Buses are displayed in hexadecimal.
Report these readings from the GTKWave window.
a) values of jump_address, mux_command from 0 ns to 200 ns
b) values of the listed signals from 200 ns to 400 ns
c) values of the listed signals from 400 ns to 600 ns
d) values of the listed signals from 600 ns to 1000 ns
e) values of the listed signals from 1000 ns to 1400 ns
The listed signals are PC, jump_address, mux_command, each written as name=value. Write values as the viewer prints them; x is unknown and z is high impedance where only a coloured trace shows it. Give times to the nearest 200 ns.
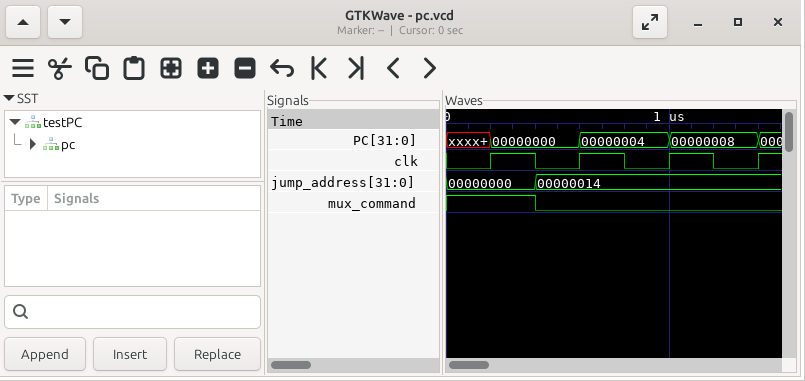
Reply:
jump_address=00000000, mux_command=1
PC=00000000, jump_address=00000000, mux_command=1
PC=00000000, jump_address=00000014, mux_command=0
PC=00000004, jump_address=00000014, mux_command=0
PC=00000008, jump_address=00000014, mux_command=0
